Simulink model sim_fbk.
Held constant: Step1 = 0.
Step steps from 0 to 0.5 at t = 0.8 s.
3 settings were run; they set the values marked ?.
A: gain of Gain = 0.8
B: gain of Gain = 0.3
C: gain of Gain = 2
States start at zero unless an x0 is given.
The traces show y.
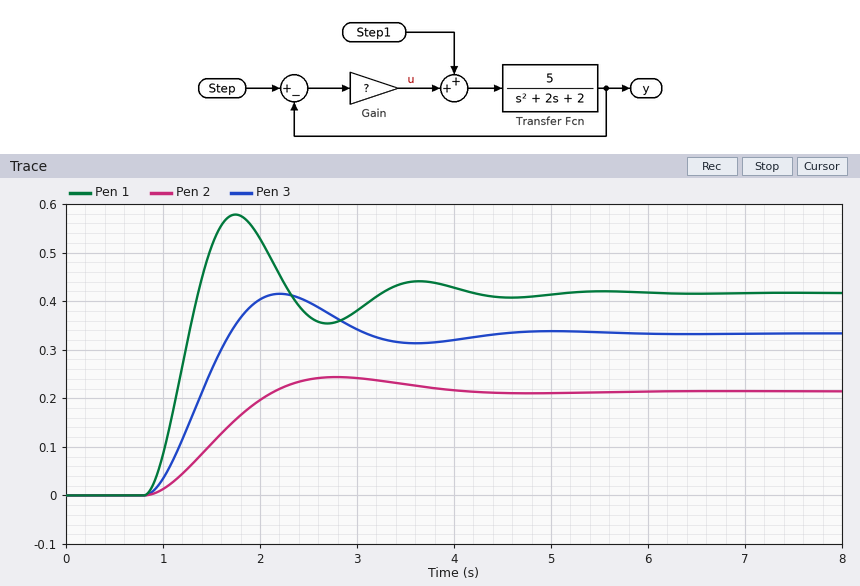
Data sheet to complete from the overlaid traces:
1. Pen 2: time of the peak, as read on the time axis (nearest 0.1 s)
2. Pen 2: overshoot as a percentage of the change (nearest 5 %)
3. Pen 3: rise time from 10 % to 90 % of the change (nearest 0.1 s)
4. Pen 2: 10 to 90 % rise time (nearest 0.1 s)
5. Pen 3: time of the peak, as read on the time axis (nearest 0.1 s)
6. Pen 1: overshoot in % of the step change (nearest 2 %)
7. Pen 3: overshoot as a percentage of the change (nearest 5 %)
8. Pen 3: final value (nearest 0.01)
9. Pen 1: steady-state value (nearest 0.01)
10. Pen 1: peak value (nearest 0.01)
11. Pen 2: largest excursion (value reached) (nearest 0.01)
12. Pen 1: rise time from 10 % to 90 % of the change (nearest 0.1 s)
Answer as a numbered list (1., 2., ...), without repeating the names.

1. 2.8 s
2. 15 %
3. 0.6 s
4. 0.9 s
5. 2.2 s
6. 38 %
7. 25 %
8. 0.33
9. 0.42
10. 0.58
11. 0.24
12. 0.4 s
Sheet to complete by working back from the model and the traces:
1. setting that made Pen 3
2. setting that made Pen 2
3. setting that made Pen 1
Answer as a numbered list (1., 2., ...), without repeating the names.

1. A
2. B
3. C
